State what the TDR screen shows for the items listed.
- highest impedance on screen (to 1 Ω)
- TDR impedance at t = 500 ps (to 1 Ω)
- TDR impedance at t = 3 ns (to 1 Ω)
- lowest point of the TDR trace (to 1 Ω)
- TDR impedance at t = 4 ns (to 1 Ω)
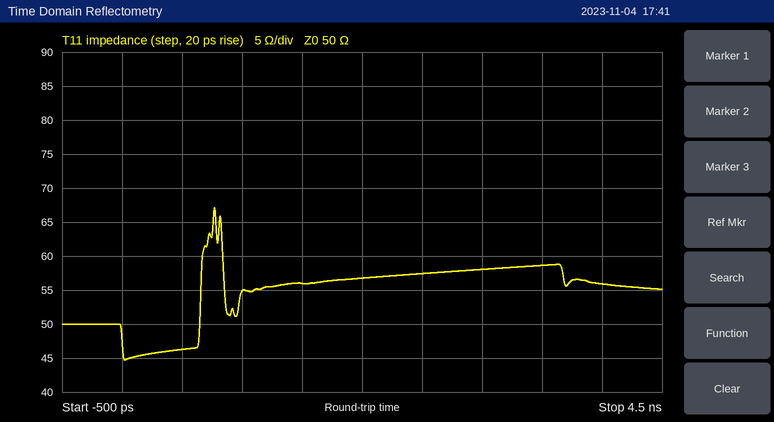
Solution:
67 Ω
46 Ω
58 Ω
45 Ω
56 Ω
